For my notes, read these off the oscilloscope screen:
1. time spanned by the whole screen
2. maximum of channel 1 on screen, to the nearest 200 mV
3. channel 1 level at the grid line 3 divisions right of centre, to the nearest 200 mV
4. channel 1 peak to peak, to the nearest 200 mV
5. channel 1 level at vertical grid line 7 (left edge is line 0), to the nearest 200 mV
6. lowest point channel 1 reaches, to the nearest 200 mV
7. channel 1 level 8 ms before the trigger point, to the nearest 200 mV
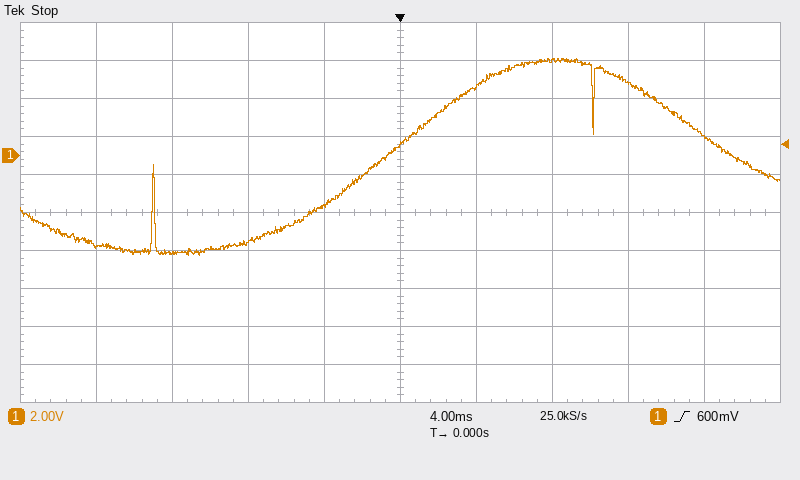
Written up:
40 ms
5.2 V
3.8 V
10.4 V
5.0 V
-5.2 V
-4.6 V
